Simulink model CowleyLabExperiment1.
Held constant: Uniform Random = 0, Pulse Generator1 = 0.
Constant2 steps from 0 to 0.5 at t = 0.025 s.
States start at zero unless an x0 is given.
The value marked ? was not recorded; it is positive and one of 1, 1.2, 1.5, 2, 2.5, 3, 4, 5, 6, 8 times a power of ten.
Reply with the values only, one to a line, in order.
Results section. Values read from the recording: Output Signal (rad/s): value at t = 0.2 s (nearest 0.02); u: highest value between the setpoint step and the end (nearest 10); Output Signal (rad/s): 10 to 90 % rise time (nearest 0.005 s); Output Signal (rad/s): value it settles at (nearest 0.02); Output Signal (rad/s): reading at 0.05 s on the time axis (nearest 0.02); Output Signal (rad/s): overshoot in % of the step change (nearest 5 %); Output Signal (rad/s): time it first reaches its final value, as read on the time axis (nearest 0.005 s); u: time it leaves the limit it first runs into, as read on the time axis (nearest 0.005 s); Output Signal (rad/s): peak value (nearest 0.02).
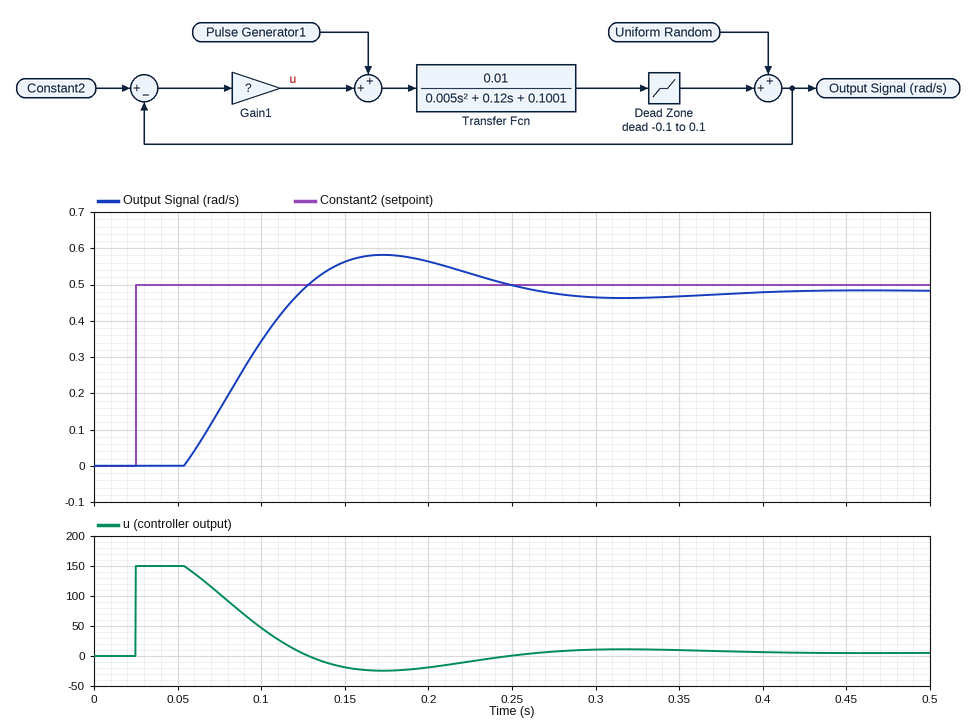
0.56
150
0.055 s
0.48
0.00
20 %
0.125 s
0.055 s
0.58
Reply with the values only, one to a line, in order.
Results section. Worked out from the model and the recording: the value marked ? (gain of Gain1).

300
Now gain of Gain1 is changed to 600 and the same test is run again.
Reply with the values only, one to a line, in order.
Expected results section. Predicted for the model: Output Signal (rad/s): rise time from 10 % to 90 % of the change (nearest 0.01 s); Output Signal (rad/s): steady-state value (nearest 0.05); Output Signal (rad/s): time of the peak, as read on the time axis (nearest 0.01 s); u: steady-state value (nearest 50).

0.03 s
0.50
0.12 s
0
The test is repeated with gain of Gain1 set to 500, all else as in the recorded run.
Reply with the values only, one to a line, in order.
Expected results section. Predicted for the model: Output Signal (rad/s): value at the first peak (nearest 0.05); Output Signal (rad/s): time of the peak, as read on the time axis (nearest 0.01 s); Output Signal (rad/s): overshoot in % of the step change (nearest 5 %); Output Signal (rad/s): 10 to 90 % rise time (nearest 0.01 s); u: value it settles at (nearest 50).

0.65
0.13 s
35 %
0.04 s
0
